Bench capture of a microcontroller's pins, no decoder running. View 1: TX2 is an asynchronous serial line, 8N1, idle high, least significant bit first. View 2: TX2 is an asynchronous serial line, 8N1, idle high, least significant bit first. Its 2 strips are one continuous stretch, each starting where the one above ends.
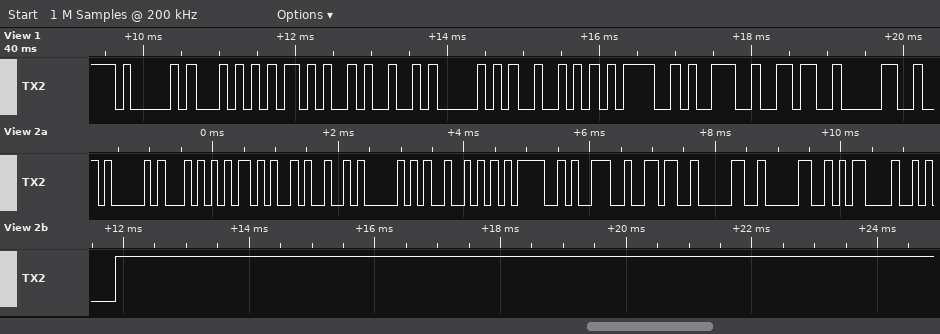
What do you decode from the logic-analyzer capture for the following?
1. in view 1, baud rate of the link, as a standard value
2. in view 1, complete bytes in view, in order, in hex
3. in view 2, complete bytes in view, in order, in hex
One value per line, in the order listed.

9600 baud
0x41 0x54 0x2B 0x49 0x50 0x52 0x3D 0x39 0x36 0x30
0x41 0x54 0x2B 0x49 0x50 0x52 0x3D 0x39 0x36 0x30 0x30 0x0D 0x0A
